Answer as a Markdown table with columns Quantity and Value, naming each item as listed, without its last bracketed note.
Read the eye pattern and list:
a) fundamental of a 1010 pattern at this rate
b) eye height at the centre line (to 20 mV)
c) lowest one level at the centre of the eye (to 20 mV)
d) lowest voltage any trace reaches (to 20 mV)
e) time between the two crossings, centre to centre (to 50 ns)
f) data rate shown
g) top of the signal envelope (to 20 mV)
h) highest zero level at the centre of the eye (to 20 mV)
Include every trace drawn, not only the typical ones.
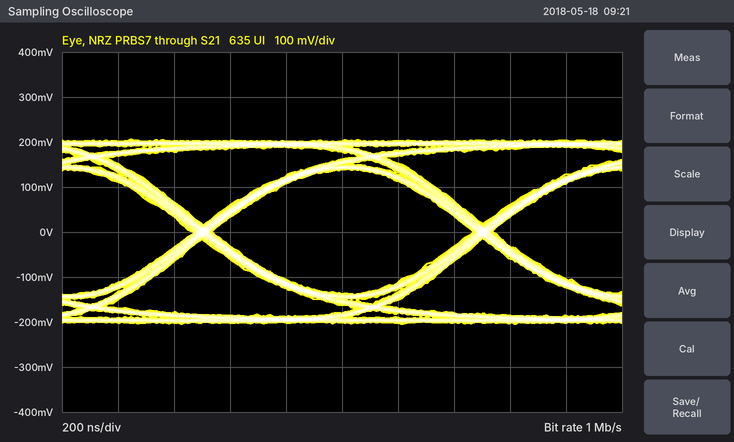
| Quantity | Value |
|---|---|
| fundamental of a 1010 pattern at this rate | 500 kHz |
| eye height at the centre line | 280 mV |
| lowest one level at the centre of the eye | 140 mV |
| lowest voltage any trace reaches | -200 mV |
| time between the two crossings, centre to centre | 1.00 µs |
| data rate shown | 1 Mb/s |
| top of the signal envelope | 200 mV |
| highest zero level at the centre of the eye | -140 mV |
